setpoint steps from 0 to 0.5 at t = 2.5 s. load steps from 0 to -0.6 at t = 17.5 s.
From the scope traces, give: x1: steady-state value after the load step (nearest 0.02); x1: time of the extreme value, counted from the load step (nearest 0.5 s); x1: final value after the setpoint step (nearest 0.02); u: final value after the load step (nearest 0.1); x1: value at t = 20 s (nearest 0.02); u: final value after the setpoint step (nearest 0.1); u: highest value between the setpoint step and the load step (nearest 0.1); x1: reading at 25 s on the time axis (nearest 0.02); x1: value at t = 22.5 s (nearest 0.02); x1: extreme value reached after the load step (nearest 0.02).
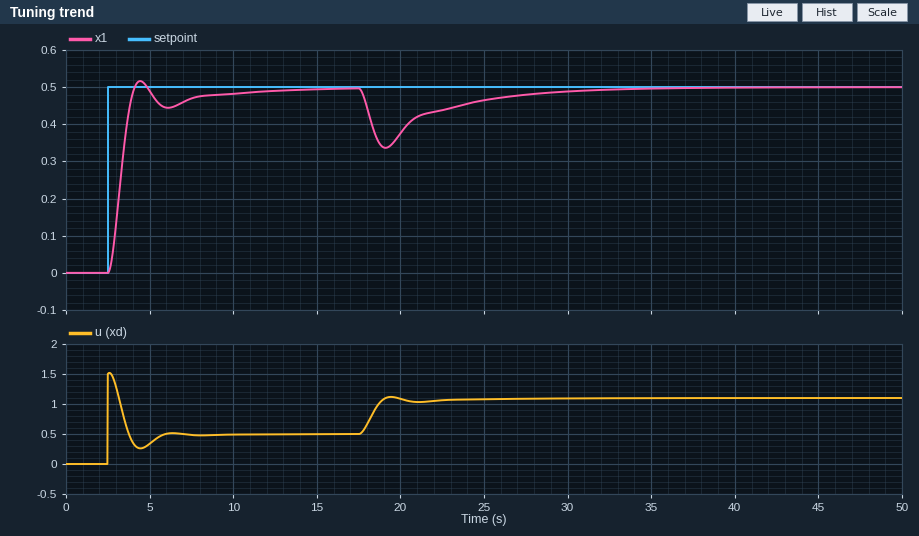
0.50
1.5 s
0.50
1.1
0.38
0.5
1.5
0.46
0.44
0.34
